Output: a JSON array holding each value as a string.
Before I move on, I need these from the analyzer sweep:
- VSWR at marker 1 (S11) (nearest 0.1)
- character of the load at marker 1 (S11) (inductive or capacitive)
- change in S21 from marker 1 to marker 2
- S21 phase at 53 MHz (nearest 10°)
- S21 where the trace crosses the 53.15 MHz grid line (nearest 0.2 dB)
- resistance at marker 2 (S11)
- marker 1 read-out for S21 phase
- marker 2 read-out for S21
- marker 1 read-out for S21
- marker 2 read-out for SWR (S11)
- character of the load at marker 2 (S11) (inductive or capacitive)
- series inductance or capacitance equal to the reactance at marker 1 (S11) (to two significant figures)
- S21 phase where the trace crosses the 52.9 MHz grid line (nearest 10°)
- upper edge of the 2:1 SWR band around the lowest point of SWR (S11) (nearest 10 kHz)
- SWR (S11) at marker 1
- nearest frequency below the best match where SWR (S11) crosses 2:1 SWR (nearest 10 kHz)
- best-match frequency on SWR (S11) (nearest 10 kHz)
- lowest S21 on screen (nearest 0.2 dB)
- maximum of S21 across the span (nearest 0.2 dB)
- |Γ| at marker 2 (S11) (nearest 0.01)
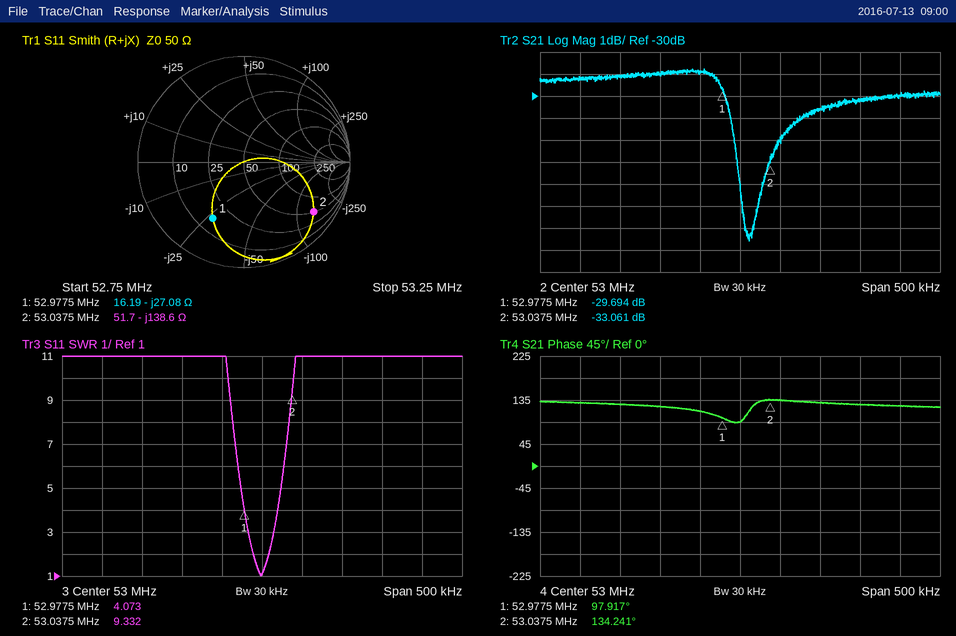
["4.1", "capacitive", "-3.367 dB", "90°", "-30.2 dB", "51.7 Ω", "97.917°", "-33.061 dB", "-29.694 dB", "9.332", "capacitive", "110 pF", "120°", "53.01 MHz", "4.073", "52.99 MHz", "53.00 MHz", "-36.6 dB", "-28.8 dB", "0.81"]
